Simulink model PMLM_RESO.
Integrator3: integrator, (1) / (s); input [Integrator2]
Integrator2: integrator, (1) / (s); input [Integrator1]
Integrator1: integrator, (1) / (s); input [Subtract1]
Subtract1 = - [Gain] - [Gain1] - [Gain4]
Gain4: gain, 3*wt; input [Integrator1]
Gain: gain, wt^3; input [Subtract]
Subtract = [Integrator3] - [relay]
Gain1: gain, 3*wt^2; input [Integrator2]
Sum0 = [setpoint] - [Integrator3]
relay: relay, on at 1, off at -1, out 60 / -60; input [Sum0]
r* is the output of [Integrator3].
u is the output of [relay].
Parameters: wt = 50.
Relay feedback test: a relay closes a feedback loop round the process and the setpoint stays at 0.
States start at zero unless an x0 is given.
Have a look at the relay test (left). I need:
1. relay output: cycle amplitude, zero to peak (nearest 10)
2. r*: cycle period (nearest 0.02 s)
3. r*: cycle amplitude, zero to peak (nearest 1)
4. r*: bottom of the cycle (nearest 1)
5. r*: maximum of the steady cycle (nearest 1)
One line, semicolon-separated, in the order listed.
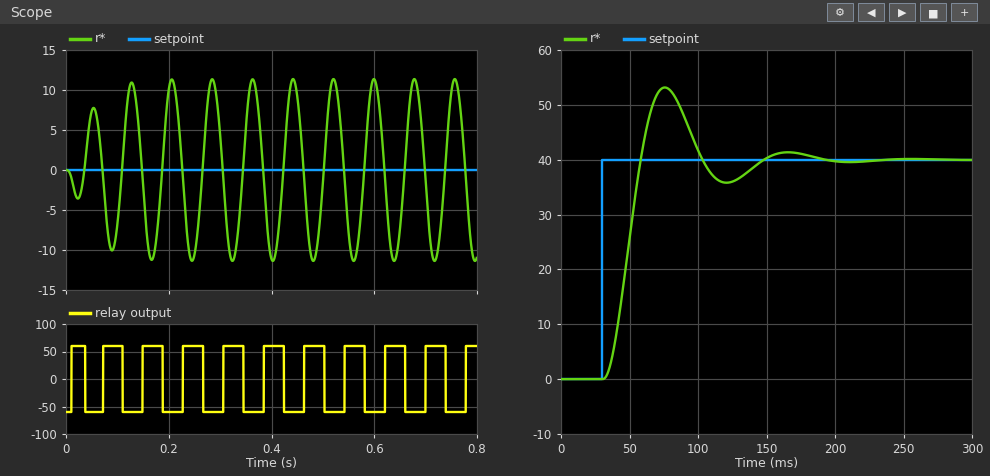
60; 0.08 s; 11; -11; 11
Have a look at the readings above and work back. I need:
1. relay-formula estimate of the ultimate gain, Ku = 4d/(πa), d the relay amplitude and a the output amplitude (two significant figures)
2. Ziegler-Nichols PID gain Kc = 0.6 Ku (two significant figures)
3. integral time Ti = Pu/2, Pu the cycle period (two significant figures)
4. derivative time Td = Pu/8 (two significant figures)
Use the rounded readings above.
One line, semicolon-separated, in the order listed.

6.9; 4.1; 0.040 s; 0.010 s
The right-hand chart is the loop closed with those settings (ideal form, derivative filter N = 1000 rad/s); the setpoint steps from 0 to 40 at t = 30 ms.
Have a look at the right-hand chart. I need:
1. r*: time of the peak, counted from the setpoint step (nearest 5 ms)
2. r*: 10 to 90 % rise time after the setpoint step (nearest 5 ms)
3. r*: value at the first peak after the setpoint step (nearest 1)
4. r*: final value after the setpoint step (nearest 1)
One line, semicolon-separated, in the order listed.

45 ms; 20 ms; 53; 40
